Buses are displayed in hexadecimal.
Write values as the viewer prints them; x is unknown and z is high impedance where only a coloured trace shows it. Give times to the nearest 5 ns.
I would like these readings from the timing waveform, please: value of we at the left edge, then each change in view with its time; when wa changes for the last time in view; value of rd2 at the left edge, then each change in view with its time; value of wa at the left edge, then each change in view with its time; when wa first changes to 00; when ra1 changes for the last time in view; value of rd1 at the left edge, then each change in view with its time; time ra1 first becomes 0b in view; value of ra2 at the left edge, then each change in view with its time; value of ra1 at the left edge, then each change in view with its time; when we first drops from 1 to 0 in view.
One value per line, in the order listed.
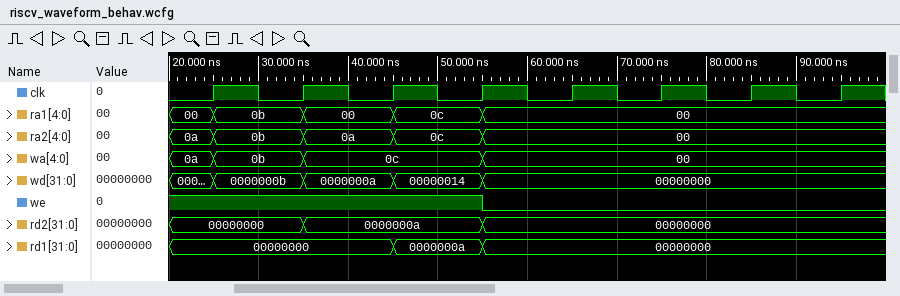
1, 0 at 55 ns
55 ns
00000000, 0000000a at 35 ns, 00000000 at 55 ns
0a, 0b at 25 ns, 0c at 35 ns, 00 at 55 ns
55 ns
55 ns
00000000, 0000000a at 45 ns, 00000000 at 55 ns
25 ns
0a, 0b at 25 ns, 0a at 35 ns, 0c at 45 ns, 00 at 55 ns
00, 0b at 25 ns, 00 at 35 ns, 0c at 45 ns, 00 at 55 ns
55 ns
